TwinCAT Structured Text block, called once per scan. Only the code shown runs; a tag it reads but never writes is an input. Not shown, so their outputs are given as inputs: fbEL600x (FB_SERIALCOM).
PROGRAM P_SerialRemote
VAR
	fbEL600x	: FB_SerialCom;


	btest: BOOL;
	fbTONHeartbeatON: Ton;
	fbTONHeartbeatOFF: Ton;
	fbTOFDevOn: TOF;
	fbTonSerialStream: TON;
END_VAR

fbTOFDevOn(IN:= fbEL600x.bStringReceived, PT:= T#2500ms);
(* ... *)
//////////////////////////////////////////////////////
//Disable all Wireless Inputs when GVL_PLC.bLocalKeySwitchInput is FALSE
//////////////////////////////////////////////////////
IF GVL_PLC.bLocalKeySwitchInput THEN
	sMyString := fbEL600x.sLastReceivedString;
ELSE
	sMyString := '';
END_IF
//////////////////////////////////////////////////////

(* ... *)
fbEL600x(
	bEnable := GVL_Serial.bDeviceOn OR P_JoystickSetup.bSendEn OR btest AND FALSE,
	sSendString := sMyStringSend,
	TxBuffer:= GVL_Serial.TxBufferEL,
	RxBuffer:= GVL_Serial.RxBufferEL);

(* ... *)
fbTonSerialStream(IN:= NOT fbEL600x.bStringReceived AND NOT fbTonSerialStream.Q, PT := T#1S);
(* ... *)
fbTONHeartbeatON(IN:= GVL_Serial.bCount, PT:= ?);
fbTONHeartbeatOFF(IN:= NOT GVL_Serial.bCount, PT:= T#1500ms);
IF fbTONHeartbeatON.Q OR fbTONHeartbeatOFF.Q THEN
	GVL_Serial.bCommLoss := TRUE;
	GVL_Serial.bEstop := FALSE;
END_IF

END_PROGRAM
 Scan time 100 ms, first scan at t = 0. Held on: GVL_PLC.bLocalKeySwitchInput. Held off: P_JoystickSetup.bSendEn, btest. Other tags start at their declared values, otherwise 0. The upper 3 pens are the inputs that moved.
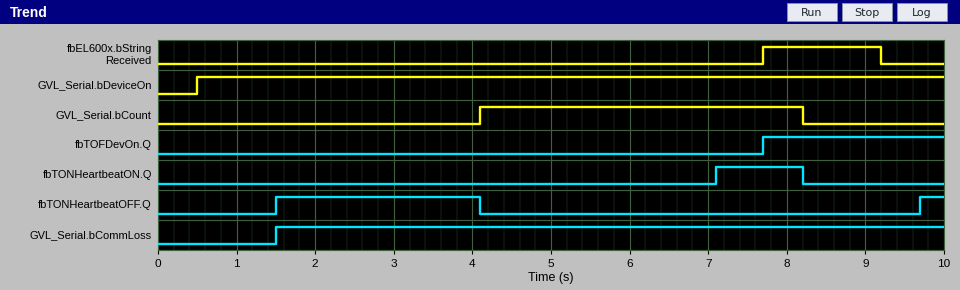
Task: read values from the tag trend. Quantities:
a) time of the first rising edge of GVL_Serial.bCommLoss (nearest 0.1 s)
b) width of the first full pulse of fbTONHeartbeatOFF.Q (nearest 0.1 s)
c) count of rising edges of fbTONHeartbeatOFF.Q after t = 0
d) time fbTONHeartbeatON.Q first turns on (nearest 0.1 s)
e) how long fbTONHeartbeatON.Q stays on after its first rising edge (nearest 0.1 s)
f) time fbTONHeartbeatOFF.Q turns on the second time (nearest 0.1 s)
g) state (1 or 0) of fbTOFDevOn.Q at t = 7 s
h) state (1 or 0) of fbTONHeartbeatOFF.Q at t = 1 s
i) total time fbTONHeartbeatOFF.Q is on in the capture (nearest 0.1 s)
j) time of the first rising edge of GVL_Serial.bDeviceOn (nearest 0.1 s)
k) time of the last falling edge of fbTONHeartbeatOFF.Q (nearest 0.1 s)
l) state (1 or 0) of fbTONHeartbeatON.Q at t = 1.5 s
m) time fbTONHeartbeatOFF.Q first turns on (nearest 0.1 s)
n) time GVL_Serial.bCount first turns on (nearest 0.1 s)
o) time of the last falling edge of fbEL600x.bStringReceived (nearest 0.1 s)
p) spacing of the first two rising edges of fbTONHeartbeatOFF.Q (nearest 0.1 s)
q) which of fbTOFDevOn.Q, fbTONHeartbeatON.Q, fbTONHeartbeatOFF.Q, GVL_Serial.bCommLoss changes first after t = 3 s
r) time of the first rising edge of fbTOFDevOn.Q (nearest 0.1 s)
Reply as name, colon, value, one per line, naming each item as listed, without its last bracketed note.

time of the first rising edge of GVL_Serial.bCommLoss: 1.5 s
width of the first full pulse of fbTONHeartbeatOFF.Q: 2.6 s
count of rising edges of fbTONHeartbeatOFF.Q after t = 0: 2
time fbTONHeartbeatON.Q first turns on: 7.1 s
how long fbTONHeartbeatON.Q stays on after its first rising edge: 1.1 s
time fbTONHeartbeatOFF.Q turns on the second time: 9.7 s
state (1 or 0) of fbTOFDevOn.Q at t = 7 s: 0
state (1 or 0) of fbTONHeartbeatOFF.Q at t = 1 s: 0
total time fbTONHeartbeatOFF.Q is on in the capture: 2.9 s
time of the first rising edge of GVL_Serial.bDeviceOn: 0.5 s
time of the last falling edge of fbTONHeartbeatOFF.Q: 4.1 s
state (1 or 0) of fbTONHeartbeatON.Q at t = 1.5 s: 0
time fbTONHeartbeatOFF.Q first turns on: 1.5 s
time GVL_Serial.bCount first turns on: 4.1 s
time of the last falling edge of fbEL600x.bStringReceived: 9.2 s
spacing of the first two rising edges of fbTONHeartbeatOFF.Q: 8.2 s
which of fbTOFDevOn.Q, fbTONHeartbeatON.Q, fbTONHeartbeatOFF.Q, GVL_Serial.bCommLoss changes first after t = 3 s: fbTONHeartbeatOFF.Q
time of the first rising edge of fbTOFDevOn.Q: 7.7 s
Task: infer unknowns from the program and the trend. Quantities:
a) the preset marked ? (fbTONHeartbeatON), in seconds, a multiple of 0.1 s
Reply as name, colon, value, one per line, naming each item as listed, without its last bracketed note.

the preset marked ? (fbTONHeartbeatON), in seconds, a multiple of 0.1 s: 3.0 s
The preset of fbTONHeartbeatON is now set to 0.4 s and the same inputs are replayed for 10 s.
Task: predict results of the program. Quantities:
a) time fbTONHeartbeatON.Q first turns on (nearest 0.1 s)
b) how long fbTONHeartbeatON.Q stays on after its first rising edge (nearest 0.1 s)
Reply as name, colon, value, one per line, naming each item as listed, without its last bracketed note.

time fbTONHeartbeatON.Q first turns on: 4.5 s
how long fbTONHeartbeatON.Q stays on after its first rising edge: 3.7 s
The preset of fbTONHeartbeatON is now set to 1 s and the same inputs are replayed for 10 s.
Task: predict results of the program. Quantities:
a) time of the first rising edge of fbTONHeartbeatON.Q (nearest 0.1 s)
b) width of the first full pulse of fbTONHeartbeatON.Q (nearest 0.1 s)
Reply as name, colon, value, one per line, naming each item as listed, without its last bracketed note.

time of the first rising edge of fbTONHeartbeatON.Q: 5.1 s
width of the first full pulse of fbTONHeartbeatON.Q: 3.1 s
